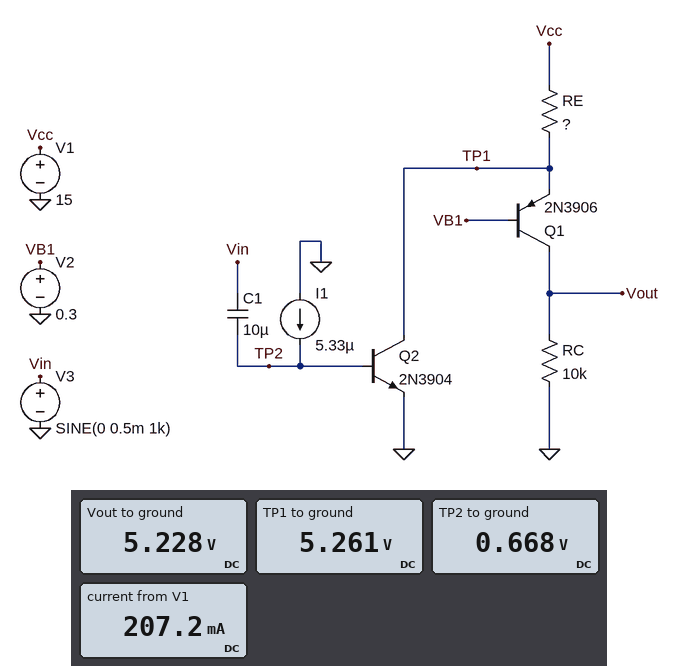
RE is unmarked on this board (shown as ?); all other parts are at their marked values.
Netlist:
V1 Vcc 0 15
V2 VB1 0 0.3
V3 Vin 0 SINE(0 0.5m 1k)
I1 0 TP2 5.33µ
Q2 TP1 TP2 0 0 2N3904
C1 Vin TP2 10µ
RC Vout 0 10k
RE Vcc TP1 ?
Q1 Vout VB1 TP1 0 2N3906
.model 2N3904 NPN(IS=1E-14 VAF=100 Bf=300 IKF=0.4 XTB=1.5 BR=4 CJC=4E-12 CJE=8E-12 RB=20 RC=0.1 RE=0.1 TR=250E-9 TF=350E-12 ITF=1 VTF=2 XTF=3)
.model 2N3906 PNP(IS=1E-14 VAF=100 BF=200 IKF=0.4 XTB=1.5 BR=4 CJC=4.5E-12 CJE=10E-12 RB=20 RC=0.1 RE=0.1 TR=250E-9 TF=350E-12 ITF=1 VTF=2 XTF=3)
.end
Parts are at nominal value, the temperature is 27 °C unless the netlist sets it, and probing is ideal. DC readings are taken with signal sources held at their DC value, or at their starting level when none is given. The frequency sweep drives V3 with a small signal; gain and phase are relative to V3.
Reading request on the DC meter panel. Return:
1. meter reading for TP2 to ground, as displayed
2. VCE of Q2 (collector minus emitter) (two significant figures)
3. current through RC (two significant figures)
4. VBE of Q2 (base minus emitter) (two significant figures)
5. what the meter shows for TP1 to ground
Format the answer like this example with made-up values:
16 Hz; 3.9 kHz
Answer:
0.668 V; 5.3 V; 520 µA; 670 mV; 5.261 V
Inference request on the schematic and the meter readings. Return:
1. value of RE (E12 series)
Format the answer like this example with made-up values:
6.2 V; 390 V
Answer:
47 Ω
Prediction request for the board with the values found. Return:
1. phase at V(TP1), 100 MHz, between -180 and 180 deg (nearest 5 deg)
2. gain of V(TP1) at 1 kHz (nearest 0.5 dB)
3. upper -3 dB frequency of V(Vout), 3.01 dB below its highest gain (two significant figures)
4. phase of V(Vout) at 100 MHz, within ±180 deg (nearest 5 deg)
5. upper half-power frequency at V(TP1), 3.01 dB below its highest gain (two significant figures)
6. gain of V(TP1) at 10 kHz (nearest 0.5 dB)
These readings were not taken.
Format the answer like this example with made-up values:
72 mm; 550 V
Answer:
150 deg; -1.0 dB; 200 MHz; 150 deg; 200 MHz; -1.0 dB
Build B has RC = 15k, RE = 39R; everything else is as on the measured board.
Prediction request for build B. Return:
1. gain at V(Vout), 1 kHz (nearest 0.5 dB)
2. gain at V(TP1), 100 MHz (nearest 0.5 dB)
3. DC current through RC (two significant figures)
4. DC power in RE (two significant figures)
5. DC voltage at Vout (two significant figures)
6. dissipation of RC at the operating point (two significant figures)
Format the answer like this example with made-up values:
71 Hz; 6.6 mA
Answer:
-1.5 dB; -2.5 dB; 390 µA; 2.2 W; 5.8 V; 2.2 mW
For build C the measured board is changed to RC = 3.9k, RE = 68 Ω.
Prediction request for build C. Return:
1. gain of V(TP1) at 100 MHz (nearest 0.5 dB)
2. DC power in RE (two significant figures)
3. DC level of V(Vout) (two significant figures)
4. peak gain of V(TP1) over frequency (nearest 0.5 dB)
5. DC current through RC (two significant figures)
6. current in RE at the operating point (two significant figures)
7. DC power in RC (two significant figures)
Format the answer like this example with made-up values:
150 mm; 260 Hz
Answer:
-1.0 dB; 1.7 W; 4.2 V; 0 dB; 1.1 mA; 160 mA; 4.6 mW
